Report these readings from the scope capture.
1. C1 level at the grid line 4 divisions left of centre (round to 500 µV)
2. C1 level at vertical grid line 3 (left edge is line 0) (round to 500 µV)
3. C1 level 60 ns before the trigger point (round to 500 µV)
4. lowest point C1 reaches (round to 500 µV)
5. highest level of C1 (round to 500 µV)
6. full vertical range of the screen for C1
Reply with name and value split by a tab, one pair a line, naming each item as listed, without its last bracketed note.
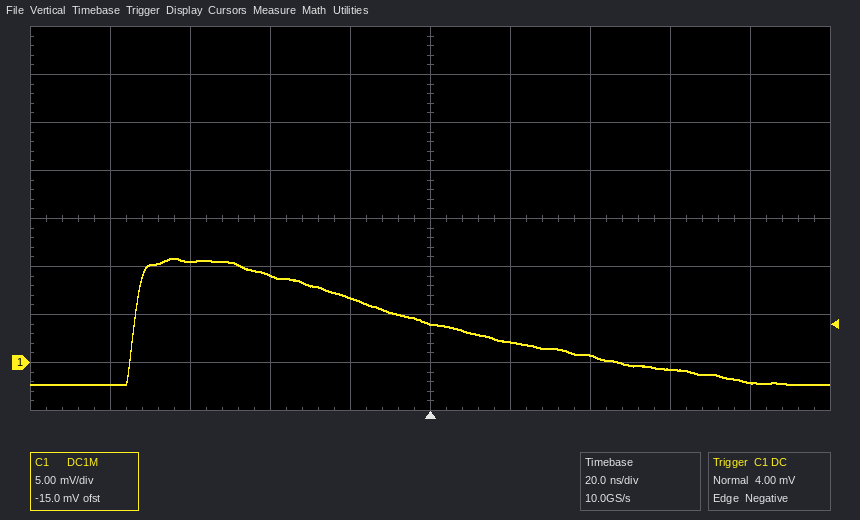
C1 level at the grid line 4 divisions left of centre	-2.5 mV
C1 level at vertical grid line 3 (left edge is line 0)	9.0 mV
C1 level 60 ns before the trigger point	10.5 mV
lowest point C1 reaches	-2.5 mV
highest level of C1	11.0 mV
full vertical range of the screen for C1	40 mV
